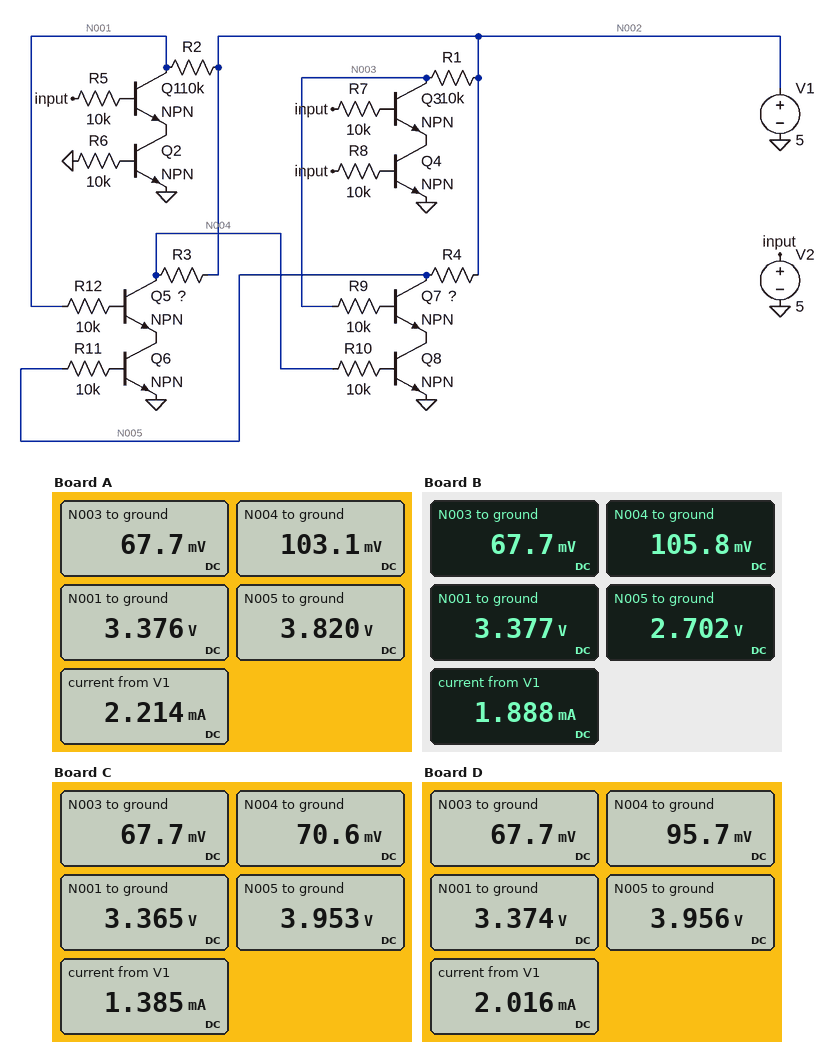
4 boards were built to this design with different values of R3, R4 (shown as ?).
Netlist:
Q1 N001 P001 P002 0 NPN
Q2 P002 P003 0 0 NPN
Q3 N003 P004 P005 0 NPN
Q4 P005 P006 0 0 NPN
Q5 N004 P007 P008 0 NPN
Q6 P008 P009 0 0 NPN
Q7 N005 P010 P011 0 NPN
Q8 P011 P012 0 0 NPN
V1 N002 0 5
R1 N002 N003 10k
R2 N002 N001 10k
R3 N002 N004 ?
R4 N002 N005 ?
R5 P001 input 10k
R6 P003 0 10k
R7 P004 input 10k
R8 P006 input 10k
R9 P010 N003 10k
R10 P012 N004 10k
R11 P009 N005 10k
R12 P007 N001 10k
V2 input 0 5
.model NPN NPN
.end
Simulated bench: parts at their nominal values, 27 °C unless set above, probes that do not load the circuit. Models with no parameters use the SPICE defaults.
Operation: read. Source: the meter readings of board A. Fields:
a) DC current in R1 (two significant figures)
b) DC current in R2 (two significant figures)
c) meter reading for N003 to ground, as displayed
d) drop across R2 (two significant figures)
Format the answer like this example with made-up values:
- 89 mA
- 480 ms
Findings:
- 490 µA
- 160 µA
- 67.7 mV
- 1.6 V
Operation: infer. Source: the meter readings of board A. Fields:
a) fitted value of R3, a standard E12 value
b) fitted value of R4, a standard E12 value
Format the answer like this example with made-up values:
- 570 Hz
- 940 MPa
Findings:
- 3.9 kΩ
- 3.9 kΩ
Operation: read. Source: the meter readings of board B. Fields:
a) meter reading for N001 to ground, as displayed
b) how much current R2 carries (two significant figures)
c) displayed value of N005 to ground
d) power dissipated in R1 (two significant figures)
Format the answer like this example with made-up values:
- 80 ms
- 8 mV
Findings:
- 3.377 V
- 160 µA
- 2.702 V
- 2.4 mW
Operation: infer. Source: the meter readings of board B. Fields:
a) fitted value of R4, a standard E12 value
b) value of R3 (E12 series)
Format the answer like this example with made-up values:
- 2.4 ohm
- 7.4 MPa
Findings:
- 12 kΩ
- 4.7 kΩ
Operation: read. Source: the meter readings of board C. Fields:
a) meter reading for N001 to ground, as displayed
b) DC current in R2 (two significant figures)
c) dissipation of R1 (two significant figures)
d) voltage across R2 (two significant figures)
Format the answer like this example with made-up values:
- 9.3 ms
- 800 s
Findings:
- 3.365 V
- 160 µA
- 2.4 mW
- 1.6 V
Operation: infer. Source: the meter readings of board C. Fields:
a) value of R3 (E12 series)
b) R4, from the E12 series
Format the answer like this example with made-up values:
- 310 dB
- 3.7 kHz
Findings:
- 12 kΩ
- 3.3 kΩ
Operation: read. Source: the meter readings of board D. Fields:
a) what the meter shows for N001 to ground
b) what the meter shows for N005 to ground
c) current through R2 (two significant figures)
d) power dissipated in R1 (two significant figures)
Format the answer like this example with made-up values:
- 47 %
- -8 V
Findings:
- 3.374 V
- 3.956 V
- 160 µA
- 2.4 mW
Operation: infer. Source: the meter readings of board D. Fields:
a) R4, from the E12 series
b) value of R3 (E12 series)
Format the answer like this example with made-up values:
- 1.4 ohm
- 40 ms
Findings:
- 3.3 kΩ
- 4.7 kΩ
